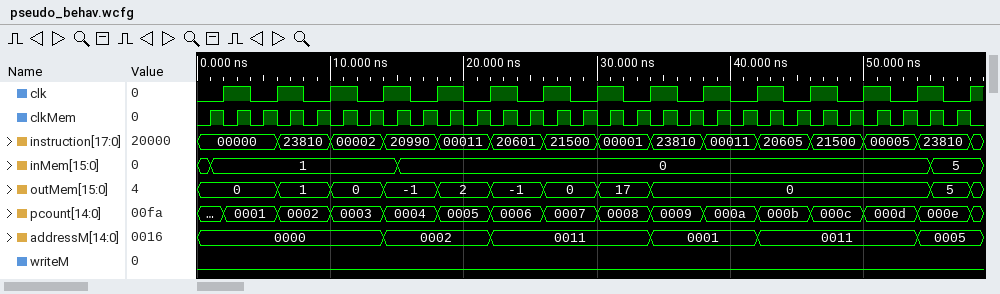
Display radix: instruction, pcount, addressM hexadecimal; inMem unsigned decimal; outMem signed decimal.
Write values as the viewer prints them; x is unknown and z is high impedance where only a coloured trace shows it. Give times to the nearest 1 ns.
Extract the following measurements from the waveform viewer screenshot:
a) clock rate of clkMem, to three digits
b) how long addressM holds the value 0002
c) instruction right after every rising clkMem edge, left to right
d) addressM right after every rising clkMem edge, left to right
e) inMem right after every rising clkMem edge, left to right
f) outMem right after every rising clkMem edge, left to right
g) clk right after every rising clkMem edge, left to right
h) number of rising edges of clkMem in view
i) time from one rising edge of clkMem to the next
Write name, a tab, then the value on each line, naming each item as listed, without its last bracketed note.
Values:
clock rate of clkMem, to three digits	500 MHz
how long addressM holds the value 0002	8 ns
instruction right after every rising clkMem edge, left to right	00000, 00000, 00000, 23810, 23810, 00002, 00002, 20990, 20990, 00011, 00011, 20601, 20601, 21500, 21500, 00001, 00001, 23810, 23810, 00011, 00011, 20605, 20605, 21500, 21500, 00005, 00005, 23810, 23810
addressM right after every rising clkMem edge, left to right	0000, 0000, 0000, 0000, 0000, 0000, 0000, 0002, 0002, 0002, 0002, 0011, 0011, 0011, 0011, 0011, 0011, 0001, 0001, 0001, 0001, 0011, 0011, 0011, 0011, 0011, 0011, 0005, 0005
inMem right after every rising clkMem edge, left to right	1, 1, 1, 1, 1, 1, 1, 0, 0, 0, 0, 0, 0, 0, 0, 0, 0, 0, 0, 0, 0, 0, 0, 0, 0, 0, 0, 5, 5
outMem right after every rising clkMem edge, left to right	0, 0, 0, 1, 1, 0, 0, -1, -1, 2, 2, -1, -1, 0, 0, 17, 17, 0, 0, 0, 0, 0, 0, 0, 0, 0, 0, 5, 5
clk right after every rising clkMem edge, left to right	0 1 0 1 0 1 0 1 0 1 0 1 0 1 0 1 0 1 0 1 0 1 0 1 0 1 0 1 0
number of rising edges of clkMem in view	29
time from one rising edge of clkMem to the next	2 ns
